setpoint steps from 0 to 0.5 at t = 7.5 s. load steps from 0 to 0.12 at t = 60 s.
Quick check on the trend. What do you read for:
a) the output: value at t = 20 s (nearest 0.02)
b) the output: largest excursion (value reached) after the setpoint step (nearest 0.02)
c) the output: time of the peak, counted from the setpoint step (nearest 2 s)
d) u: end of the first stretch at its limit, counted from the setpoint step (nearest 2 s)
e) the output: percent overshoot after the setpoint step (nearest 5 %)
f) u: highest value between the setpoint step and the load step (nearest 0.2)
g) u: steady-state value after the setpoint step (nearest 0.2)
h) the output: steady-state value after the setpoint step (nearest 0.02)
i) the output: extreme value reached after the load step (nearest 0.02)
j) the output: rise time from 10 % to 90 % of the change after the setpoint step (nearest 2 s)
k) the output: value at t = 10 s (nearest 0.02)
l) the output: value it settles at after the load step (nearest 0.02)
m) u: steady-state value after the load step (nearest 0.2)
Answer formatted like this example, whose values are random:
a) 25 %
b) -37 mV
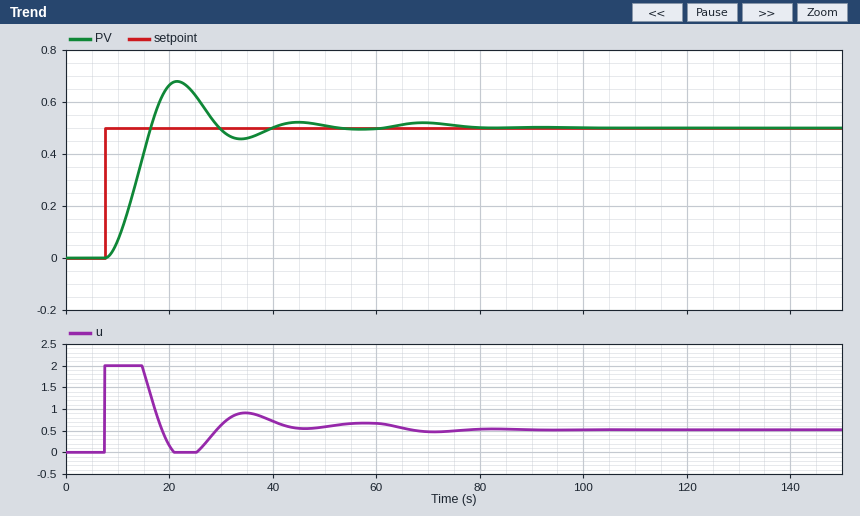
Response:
a) 0.66
b) 0.68
c) 14 s
d) 8 s
e) 35 %
f) 2.0
g) 0.6
h) 0.50
i) 0.52
j) 6 s
k) 0.06
l) 0.50
m) 0.6
